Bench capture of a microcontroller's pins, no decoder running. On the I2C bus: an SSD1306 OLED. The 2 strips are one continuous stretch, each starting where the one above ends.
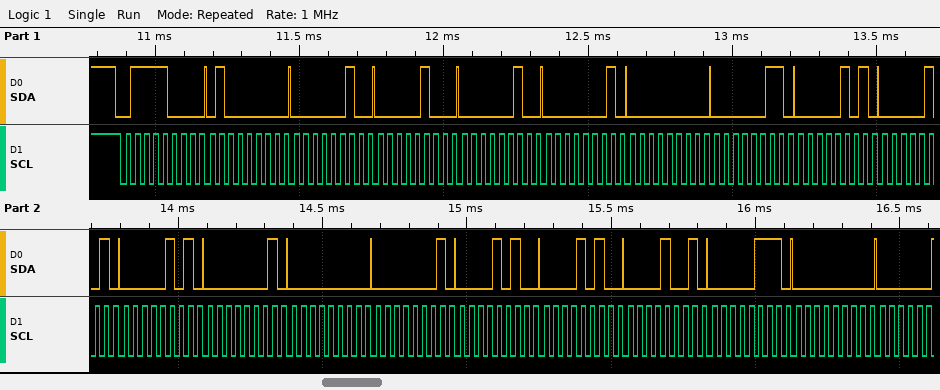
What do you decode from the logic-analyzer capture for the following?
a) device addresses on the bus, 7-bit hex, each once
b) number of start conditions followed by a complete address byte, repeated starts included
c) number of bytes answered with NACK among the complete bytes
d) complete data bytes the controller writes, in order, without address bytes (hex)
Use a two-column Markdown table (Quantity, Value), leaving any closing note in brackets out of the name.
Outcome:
| Quantity | Value |
|---|---|
| device addresses on the bus, 7-bit hex, each once | 0x3C |
| number of start conditions followed by a complete address byte, repeated starts included | 1 |
| number of bytes answered with NACK among the complete bytes | 0 |
| complete data bytes the controller writes, in order, without address bytes | 40 02 04 02 01 00 03 05 05 05 01 00 01 0A 0A 09 07 00 |
